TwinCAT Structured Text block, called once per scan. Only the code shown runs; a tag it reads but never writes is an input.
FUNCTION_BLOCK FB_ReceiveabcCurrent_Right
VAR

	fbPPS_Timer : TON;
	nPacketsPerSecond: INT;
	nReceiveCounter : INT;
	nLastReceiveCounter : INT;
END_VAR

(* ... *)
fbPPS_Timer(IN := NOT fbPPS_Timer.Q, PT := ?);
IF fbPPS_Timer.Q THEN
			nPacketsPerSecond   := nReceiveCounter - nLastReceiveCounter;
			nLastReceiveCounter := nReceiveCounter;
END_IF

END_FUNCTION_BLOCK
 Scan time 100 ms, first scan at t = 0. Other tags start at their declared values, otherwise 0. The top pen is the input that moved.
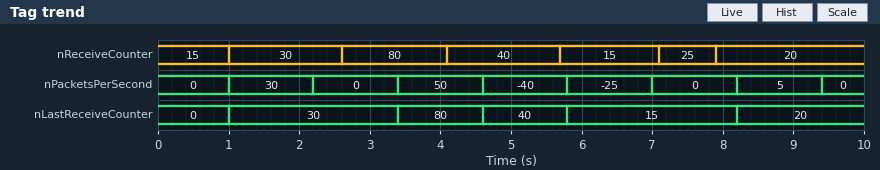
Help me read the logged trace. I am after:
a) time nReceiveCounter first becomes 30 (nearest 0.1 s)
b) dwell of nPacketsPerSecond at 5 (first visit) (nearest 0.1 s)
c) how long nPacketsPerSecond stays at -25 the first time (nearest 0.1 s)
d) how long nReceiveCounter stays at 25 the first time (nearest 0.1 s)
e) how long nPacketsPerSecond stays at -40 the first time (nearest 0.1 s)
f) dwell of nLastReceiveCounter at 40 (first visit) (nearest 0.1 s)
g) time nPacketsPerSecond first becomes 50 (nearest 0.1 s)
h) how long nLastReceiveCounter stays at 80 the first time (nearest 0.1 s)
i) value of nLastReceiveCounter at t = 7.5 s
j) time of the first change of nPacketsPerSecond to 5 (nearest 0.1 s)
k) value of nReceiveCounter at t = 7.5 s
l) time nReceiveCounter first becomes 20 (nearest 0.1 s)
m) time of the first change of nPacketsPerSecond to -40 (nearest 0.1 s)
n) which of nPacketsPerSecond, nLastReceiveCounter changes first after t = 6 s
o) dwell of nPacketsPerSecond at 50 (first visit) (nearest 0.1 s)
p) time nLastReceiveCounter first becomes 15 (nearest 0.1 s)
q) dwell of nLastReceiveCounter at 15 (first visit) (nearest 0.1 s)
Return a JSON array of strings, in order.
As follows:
["1.0 s", "1.2 s", "1.2 s", "0.8 s", "1.2 s", "1.2 s", "3.4 s", "1.2 s", "15", "8.2 s", "25", "7.9 s", "4.6 s", "nPacketsPerSecond", "1.2 s", "5.8 s", "2.4 s"]
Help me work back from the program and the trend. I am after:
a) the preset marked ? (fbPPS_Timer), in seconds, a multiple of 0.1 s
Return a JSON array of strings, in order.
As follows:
["1.0 s"]
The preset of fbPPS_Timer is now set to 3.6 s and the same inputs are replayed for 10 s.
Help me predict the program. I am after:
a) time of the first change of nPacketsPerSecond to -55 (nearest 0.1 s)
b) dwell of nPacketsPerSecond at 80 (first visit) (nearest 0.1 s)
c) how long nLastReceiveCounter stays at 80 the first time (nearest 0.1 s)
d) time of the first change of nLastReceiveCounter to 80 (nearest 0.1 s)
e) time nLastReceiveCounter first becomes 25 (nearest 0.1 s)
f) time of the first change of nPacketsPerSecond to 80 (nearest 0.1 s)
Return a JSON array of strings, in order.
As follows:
["7.4 s", "3.8 s", "3.8 s", "3.6 s", "7.4 s", "3.6 s"]
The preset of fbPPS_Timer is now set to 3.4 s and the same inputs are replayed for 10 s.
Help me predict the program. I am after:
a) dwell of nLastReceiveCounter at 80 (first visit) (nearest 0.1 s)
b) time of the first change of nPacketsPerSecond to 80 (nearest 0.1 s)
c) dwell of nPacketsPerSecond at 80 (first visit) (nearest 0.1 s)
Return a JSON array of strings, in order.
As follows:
["3.6 s", "3.4 s", "3.6 s"]
